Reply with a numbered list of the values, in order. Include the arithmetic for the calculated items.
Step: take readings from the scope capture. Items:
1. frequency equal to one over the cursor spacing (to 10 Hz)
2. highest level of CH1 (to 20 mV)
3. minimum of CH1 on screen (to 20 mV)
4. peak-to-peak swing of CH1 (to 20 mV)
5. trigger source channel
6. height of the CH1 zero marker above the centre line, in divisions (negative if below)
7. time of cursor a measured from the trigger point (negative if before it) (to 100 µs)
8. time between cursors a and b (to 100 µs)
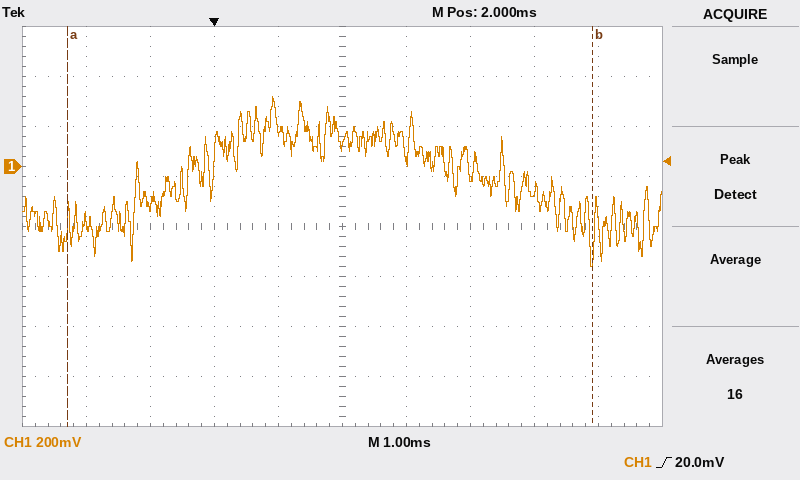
1. 1 / 8.2 ms ≈ 120 Hz
2. 280 mV
3. -400 mV
4. 280 mV − (-400 mV) = 680 mV
5. CH1
6. +1.2 div
7. -2.3 ms
8. 8.2 ms
